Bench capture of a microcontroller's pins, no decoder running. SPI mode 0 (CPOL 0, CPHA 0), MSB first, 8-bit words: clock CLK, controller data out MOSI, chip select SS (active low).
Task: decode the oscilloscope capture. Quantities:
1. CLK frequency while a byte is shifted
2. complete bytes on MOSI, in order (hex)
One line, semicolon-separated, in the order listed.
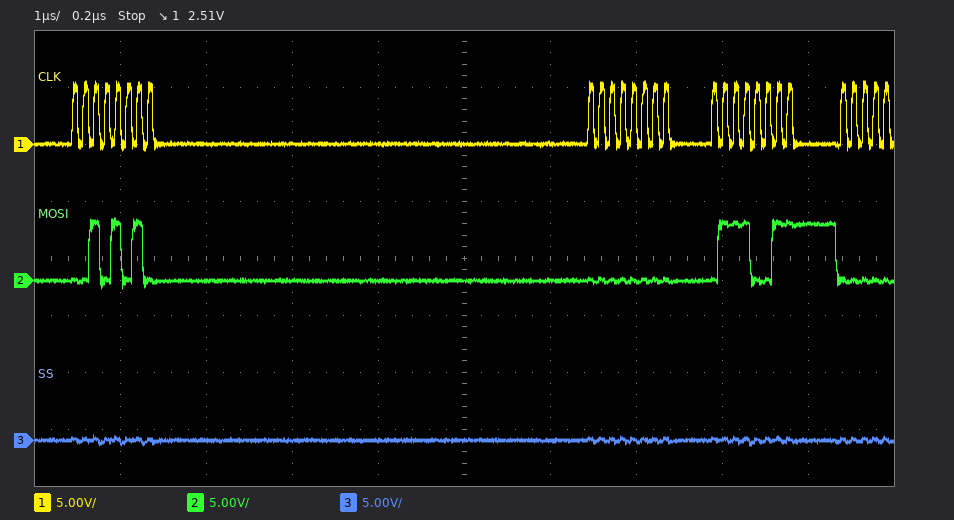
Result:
8 MHz; 2A 00 73
